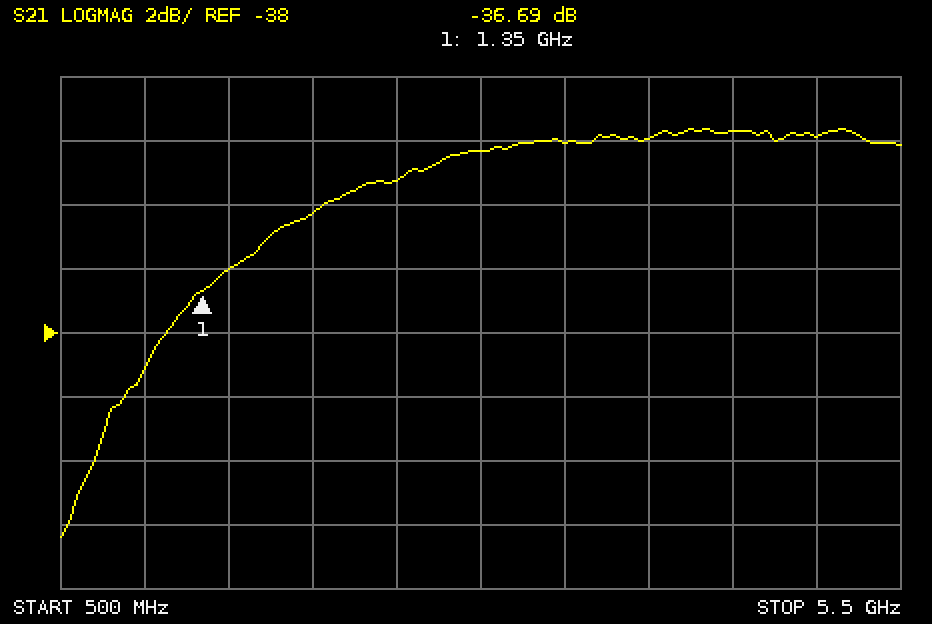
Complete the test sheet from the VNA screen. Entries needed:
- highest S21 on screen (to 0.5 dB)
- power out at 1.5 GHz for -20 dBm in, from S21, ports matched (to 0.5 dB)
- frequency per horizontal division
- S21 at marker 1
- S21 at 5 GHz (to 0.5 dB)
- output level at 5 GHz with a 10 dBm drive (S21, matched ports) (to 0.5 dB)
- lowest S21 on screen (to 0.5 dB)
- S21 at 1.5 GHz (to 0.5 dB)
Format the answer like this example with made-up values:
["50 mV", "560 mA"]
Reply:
["-31.5 dB", "-56.0 dBm", "500 MHz", "-36.69 dB", "-32.0 dB", "-22.0 dBm", "-44.5 dB", "-36.0 dB"]
